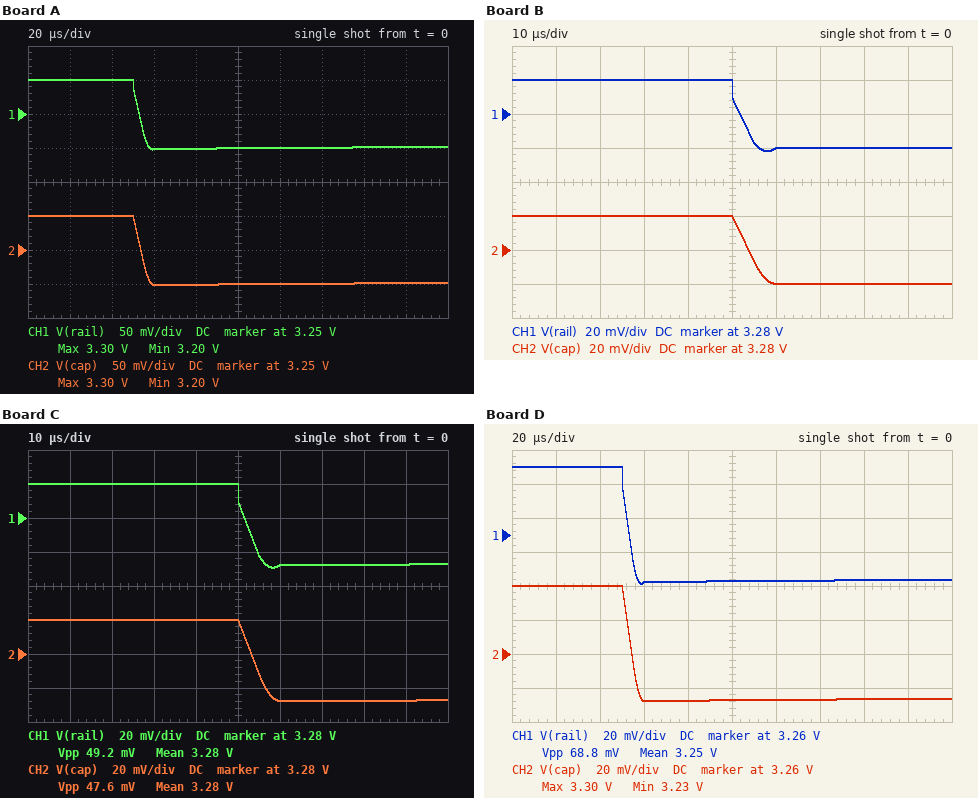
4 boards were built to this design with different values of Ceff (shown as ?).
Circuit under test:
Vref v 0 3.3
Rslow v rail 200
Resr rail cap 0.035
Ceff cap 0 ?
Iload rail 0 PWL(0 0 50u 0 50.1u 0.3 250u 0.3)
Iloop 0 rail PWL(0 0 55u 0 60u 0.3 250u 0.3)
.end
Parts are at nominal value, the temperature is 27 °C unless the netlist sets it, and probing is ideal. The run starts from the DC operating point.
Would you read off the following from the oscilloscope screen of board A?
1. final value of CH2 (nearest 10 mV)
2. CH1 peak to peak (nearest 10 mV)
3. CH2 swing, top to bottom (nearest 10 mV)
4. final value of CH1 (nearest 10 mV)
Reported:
3.20 V
100 mV
100 mV
3.20 V
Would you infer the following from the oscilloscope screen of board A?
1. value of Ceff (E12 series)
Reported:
22 µF
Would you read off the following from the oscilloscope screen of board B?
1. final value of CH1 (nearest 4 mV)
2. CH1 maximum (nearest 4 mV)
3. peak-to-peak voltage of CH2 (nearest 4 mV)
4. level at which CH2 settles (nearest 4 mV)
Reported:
3.260 V
3.300 V
40 mV
3.260 V
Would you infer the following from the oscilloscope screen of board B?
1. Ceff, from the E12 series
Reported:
56 µF
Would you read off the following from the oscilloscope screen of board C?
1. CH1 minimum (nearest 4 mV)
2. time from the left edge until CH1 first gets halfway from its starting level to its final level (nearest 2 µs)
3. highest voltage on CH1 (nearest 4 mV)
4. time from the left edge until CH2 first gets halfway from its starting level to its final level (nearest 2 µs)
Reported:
3.252 V
52 µs
3.300 V
54 µs
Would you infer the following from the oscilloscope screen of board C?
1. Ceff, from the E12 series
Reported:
47 µF
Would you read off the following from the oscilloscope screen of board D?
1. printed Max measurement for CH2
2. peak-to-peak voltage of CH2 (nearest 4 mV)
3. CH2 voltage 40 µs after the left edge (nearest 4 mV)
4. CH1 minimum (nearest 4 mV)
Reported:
3.30 V
68 mV
3.300 V
3.232 V
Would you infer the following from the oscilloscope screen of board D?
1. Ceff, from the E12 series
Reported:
33 µF
